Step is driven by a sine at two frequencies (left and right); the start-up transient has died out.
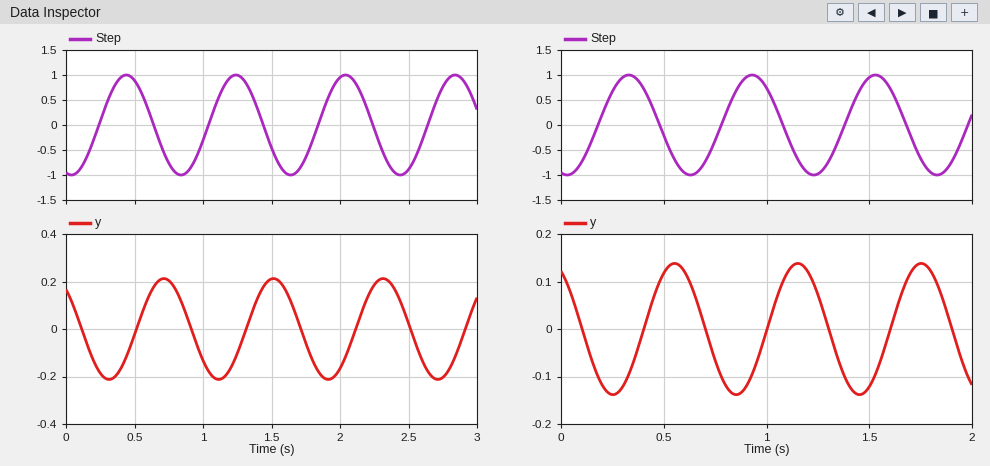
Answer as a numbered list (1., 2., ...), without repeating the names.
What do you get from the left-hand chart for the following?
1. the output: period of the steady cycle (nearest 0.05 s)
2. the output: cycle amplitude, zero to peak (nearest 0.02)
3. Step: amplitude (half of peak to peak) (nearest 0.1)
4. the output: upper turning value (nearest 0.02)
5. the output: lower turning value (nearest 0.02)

1. 0.80 s
2. 0.22
3. 1.0
4. 0.22
5. -0.22
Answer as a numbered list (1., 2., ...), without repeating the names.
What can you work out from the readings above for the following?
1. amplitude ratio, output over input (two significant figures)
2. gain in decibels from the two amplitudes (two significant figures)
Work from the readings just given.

1. 0.22
2. -13 dB
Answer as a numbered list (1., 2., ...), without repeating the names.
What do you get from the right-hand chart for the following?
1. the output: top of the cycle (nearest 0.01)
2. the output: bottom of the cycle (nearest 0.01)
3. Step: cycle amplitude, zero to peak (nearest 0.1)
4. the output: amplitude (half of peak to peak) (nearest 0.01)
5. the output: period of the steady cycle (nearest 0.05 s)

1. 0.14
2. -0.14
3. 1.0
4. 0.14
5. 0.60 s
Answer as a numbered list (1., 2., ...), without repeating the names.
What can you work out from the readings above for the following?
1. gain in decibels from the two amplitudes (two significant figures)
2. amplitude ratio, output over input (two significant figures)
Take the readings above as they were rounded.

1. -17 dB
2. 0.14
